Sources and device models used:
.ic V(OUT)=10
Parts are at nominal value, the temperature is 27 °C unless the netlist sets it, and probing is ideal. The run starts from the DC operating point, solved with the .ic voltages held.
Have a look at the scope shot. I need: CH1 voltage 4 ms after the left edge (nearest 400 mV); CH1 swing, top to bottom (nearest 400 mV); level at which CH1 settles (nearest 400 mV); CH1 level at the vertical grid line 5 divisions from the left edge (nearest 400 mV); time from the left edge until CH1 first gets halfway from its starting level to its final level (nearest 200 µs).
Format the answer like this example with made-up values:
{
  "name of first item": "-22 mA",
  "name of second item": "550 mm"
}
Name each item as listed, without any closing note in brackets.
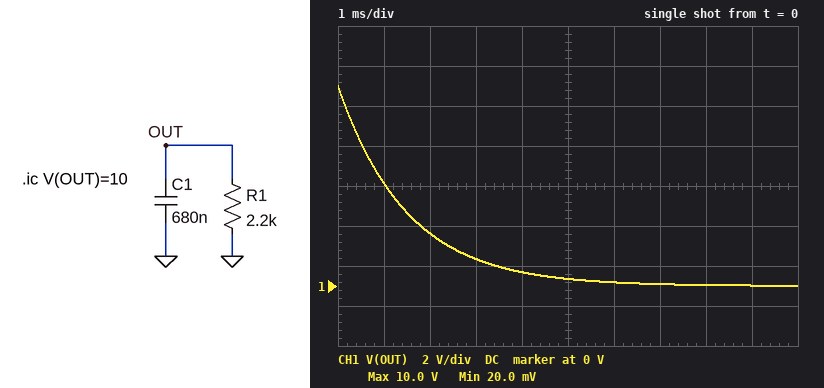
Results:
{
  "CH1 voltage 4 ms after the left edge": "800 mV",
  "CH1 swing, top to bottom": "10.0 V",
  "level at which CH1 settles": "0 V",
  "CH1 level at the vertical grid line 5 divisions from the left edge": "400 mV",
  "time from the left edge until CH1 first gets halfway from its starting level to its final level": "1.0 ms"
}
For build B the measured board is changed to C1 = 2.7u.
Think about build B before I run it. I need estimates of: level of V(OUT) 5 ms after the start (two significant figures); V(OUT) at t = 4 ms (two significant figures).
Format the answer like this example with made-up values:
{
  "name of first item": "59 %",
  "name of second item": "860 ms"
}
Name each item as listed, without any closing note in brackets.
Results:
{
  "level of V(OUT) 5 ms after the start": "4.3 V",
  "V(OUT) at t = 4 ms": "5.1 V"
}
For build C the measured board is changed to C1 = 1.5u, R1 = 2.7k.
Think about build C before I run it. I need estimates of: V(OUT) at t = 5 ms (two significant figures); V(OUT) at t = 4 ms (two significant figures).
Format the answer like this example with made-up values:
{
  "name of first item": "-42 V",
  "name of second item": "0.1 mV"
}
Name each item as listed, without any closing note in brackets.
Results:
{
  "V(OUT) at t = 5 ms": "2.9 V",
  "V(OUT) at t = 4 ms": "3.7 V"
}
